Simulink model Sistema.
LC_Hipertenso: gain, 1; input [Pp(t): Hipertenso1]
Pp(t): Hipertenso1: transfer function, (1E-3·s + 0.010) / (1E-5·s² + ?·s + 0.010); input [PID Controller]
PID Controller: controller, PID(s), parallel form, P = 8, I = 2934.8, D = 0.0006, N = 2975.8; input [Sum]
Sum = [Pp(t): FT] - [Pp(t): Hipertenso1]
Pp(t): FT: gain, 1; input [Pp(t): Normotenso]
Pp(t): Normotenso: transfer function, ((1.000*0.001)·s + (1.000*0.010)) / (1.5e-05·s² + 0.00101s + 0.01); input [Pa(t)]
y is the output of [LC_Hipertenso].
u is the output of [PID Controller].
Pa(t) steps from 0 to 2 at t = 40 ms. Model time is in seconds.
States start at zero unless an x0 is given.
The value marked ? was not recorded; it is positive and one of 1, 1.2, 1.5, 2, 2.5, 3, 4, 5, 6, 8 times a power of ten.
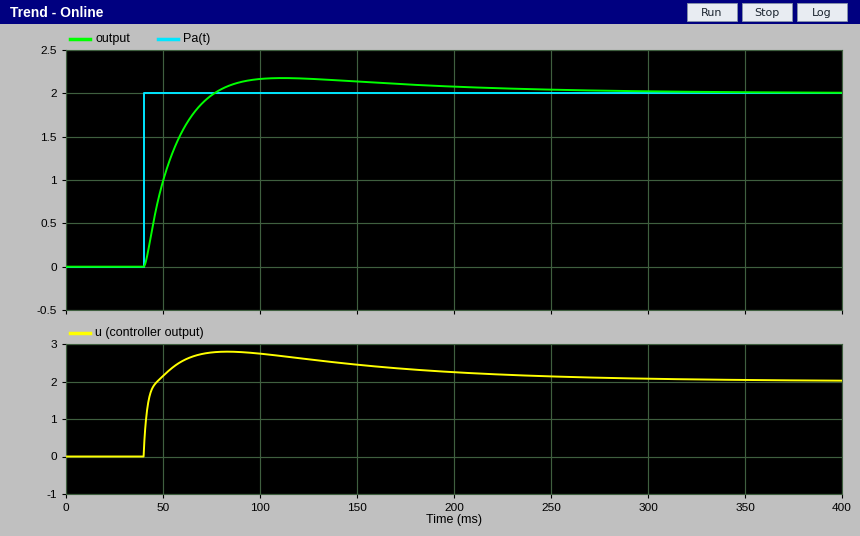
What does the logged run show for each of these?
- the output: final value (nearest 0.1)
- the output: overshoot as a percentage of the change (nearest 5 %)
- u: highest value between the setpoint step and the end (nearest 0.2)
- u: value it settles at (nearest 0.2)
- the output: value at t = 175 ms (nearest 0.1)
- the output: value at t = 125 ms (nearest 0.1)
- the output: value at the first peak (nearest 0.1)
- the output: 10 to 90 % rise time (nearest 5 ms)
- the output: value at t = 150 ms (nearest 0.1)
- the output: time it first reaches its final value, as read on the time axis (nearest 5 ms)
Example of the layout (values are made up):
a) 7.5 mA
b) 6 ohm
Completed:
a) 2.0
b) 10 %
c) 2.8
d) 2.0
e) 2.1
f) 2.2
g) 2.2
h) 25 ms
i) 2.1
j) 75 ms
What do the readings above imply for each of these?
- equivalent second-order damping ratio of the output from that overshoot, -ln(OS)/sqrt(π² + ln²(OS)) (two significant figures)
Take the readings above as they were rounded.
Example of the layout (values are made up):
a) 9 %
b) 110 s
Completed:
a) 0.59
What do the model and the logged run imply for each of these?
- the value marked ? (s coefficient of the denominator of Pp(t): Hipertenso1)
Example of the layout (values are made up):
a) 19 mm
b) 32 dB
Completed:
a) 0.0015
